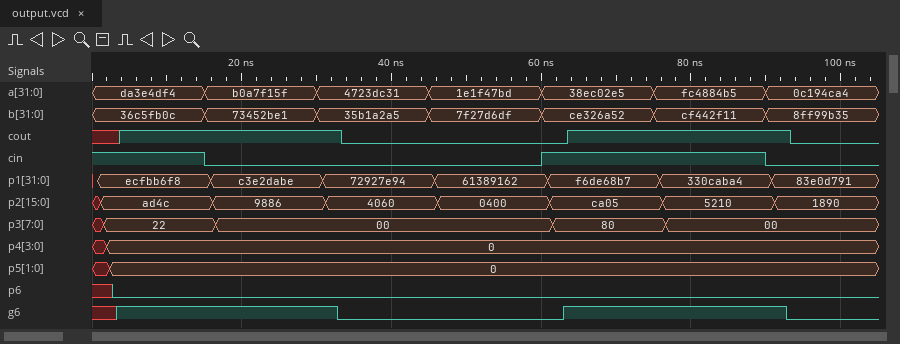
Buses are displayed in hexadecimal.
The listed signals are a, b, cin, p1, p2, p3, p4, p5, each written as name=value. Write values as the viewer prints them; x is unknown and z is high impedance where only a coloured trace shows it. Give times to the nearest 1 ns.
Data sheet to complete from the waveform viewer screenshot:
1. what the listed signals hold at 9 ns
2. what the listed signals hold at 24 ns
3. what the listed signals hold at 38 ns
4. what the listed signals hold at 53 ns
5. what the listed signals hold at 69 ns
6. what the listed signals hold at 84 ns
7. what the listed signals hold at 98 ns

a=da3e4df4, b=36c5fb0c, cin=1, p1=ecfbb6f8, p2=ad4c, p3=22, p4=0, p5=0
a=b0a7f15f, b=73452be1, cin=0, p1=c3e2dabe, p2=9886, p3=00, p4=0, p5=0
a=4723dc31, b=35b1a2a5, cin=0, p1=72927e94, p2=4060, p3=00, p4=0, p5=0
a=1e1f47bd, b=7f27d6df, cin=0, p1=61389162, p2=0400, p3=00, p4=0, p5=0
a=38ec02e5, b=ce326a52, cin=1, p1=f6de68b7, p2=ca05, p3=80, p4=0, p5=0
a=fc4884b5, b=cf442f11, cin=1, p1=330caba4, p2=5210, p3=00, p4=0, p5=0
a=0c194ca4, b=8ff99b35, cin=0, p1=83e0d791, p2=1890, p3=00, p4=0, p5=0
